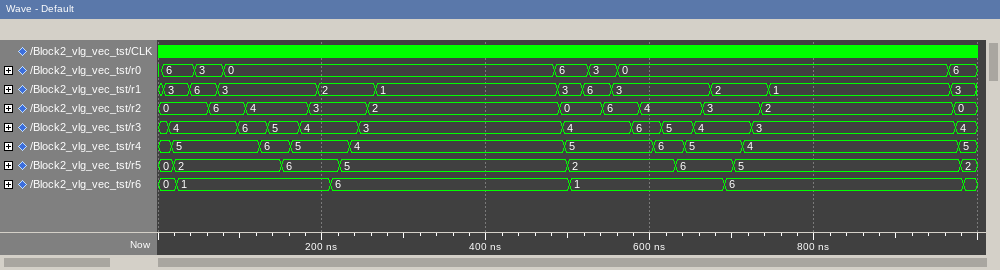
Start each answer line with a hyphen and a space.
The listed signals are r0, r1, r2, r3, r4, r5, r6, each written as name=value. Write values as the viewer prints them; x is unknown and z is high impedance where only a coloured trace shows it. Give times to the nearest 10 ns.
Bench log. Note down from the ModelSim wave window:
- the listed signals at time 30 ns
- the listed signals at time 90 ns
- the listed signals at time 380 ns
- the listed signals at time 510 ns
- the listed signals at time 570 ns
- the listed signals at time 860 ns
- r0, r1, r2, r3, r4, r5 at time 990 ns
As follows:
- r0=6, r1=3, r2=0, r3=4, r4=5, r5=2, r6=1
- r0=0, r1=3, r2=6, r3=4, r4=5, r5=2, r6=1
- r0=0, r1=1, r2=2, r3=3, r4=4, r5=5, r6=6
- r0=6, r1=3, r2=0, r3=4, r4=5, r5=2, r6=1
- r0=0, r1=3, r2=6, r3=4, r4=5, r5=2, r6=1
- r0=0, r1=1, r2=2, r3=3, r4=4, r5=5, r6=6
- r0=6, r1=3, r2=0, r3=4, r4=5, r5=2
